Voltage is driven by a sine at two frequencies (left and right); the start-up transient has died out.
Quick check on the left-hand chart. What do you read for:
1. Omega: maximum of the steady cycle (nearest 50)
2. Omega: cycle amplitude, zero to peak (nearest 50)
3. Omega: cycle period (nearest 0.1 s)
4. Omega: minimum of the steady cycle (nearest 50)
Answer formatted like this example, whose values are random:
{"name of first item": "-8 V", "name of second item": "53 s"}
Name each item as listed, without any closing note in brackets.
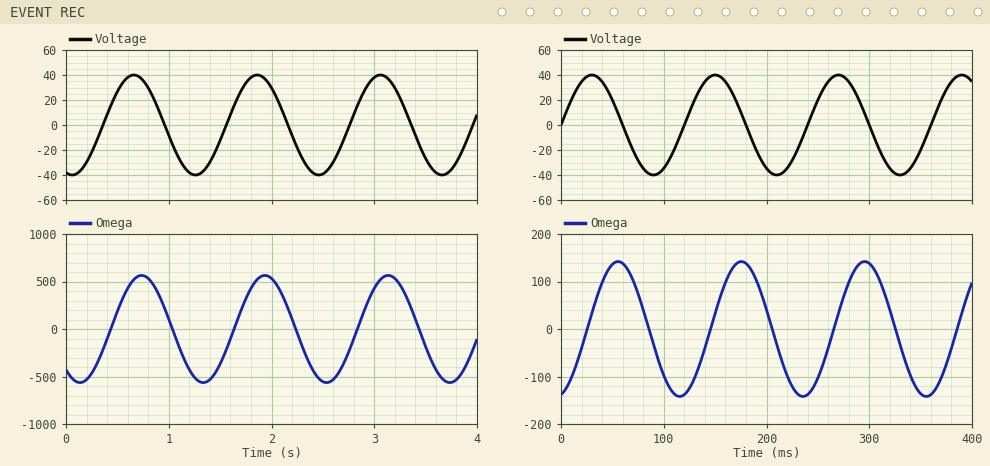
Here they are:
{"Omega: maximum of the steady cycle": "550", "Omega: cycle amplitude, zero to peak": "550", "Omega: cycle period": "1.2 s", "Omega: minimum of the steady cycle": "-550"}
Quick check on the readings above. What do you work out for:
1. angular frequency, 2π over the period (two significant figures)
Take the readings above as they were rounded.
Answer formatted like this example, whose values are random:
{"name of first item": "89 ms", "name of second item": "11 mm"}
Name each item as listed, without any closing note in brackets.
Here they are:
{"angular frequency, 2π over the period": "5.2 rad/s"}
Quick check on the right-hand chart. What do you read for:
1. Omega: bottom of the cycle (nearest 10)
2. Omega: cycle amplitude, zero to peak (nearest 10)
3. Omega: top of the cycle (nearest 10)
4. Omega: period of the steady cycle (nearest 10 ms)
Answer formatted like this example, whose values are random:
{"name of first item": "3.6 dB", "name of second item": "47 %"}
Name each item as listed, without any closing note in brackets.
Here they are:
{"Omega: bottom of the cycle": "-140", "Omega: cycle amplitude, zero to peak": "140", "Omega: top of the cycle": "140", "Omega: period of the steady cycle": "120 ms"}
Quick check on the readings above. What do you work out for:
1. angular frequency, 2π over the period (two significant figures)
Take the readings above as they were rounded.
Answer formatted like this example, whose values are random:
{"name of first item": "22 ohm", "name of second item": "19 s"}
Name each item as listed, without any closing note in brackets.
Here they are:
{"angular frequency, 2π over the period": "0.052 rad/ms"}
